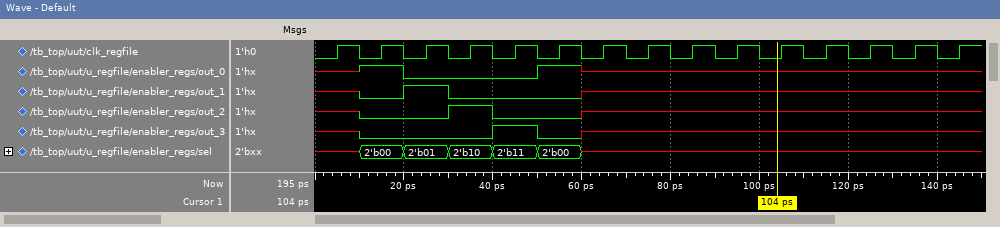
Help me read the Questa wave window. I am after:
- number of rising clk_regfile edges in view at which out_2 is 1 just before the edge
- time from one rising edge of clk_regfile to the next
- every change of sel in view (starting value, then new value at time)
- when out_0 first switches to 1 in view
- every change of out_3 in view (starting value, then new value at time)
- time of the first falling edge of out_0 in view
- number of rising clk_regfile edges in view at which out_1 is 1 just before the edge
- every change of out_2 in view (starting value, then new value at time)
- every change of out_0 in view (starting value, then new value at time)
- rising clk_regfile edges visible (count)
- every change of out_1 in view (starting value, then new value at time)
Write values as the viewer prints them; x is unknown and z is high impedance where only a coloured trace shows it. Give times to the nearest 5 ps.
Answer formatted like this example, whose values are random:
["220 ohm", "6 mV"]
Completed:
["1", "10 ps", "x, 2'b00 at 10 ps, 2'b01 at 20 ps, 2'b10 at 30 ps, 2'b11 at 40 ps, 2'b00 at 50 ps, x at 60 ps", "10 ps", "x, 0 at 10 ps, 1 at 40 ps, 0 at 50 ps, x at 60 ps", "20 ps", "1", "x, 0 at 10 ps, 1 at 30 ps, 0 at 40 ps, x at 60 ps", "x, 1 at 10 ps, 0 at 20 ps, 1 at 50 ps, x at 60 ps", "15", "x, 0 at 10 ps, 1 at 20 ps, 0 at 30 ps, x at 60 ps"]
